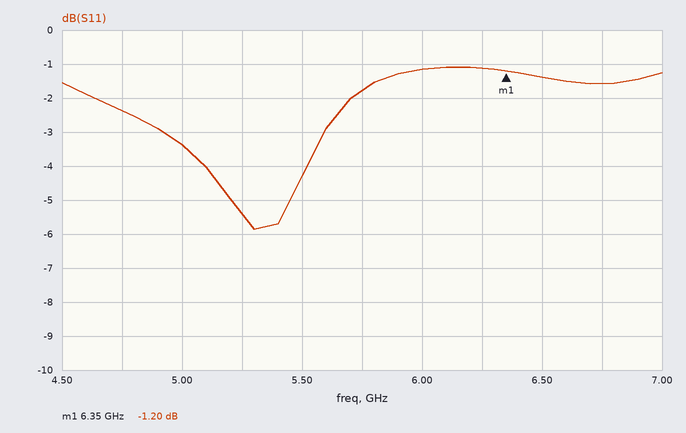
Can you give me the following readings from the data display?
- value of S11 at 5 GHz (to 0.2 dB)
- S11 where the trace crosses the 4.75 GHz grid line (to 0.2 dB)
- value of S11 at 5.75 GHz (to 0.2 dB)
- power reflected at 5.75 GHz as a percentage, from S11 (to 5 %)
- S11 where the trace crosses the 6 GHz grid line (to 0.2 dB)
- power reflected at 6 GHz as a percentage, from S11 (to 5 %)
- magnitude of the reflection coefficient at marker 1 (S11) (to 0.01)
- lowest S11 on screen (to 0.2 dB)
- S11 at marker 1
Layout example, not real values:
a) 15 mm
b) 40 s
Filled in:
a) -3.4 dB
b) -2.4 dB
c) -1.8 dB
d) 65 %
e) -1.2 dB
f) 75 %
g) 0.87
h) -5.8 dB
i) -1.20 dB
